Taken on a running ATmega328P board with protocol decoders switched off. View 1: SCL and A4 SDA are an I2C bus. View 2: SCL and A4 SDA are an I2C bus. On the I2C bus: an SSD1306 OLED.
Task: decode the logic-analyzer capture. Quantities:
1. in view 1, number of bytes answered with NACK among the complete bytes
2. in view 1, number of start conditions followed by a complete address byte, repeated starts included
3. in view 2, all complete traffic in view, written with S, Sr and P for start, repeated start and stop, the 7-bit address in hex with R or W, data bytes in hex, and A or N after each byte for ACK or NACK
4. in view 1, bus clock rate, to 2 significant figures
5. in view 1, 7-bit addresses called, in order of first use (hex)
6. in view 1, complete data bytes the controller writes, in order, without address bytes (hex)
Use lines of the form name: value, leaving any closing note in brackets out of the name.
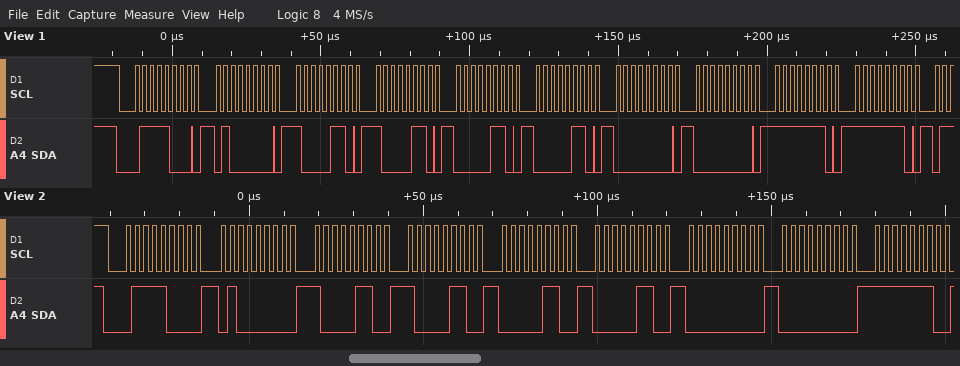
in view 1, number of bytes answered with NACK among the complete bytes: 0
in view 1, number of start conditions followed by a complete address byte, repeated starts included: 1
in view 2, all complete traffic in view, written with S, Sr and P for start, repeated start and stop, the 7-bit address in hex with R or W, data bytes in hex, and A or N after each byte for ACK or NACK: S 3CW A 40 A 86 A 86 A 06 A 06 A 00 A 00 A FE A
in view 1, bus clock rate, to 2 significant figures: 400 kHz
in view 1, 7-bit addresses called, in order of first use: 0x3C
in view 1, complete data bytes the controller writes, in order, without address bytes: 40 86 86 06 06 00 00 FE FE
